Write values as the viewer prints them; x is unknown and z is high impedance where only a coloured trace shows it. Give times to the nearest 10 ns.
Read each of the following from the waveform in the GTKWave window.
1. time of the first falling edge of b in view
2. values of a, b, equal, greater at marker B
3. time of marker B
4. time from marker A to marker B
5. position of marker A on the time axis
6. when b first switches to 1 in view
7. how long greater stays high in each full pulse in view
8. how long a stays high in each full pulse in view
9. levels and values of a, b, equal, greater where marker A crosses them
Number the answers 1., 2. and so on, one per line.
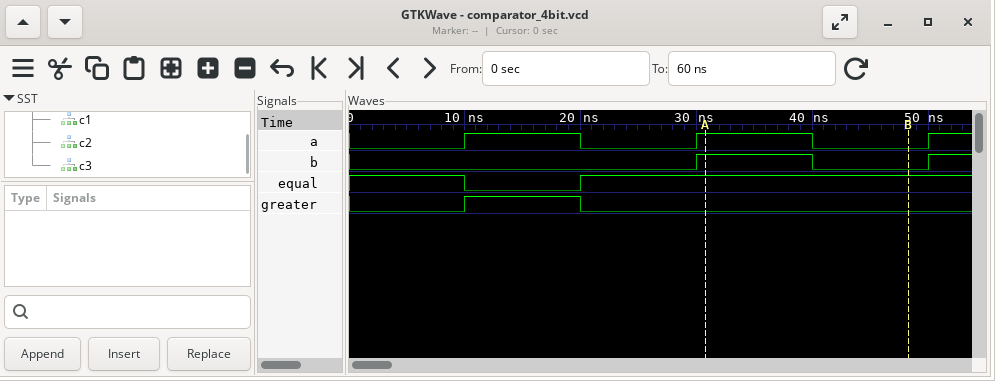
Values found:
1. 40 ns
2. a=0, b=0, equal=1, greater=0
3. 50 ns
4. 20 ns
5. 30 ns
6. 30 ns
7. 10 ns
8. 10 ns, 10 ns
9. a=1, b=1, equal=1, greater=0
